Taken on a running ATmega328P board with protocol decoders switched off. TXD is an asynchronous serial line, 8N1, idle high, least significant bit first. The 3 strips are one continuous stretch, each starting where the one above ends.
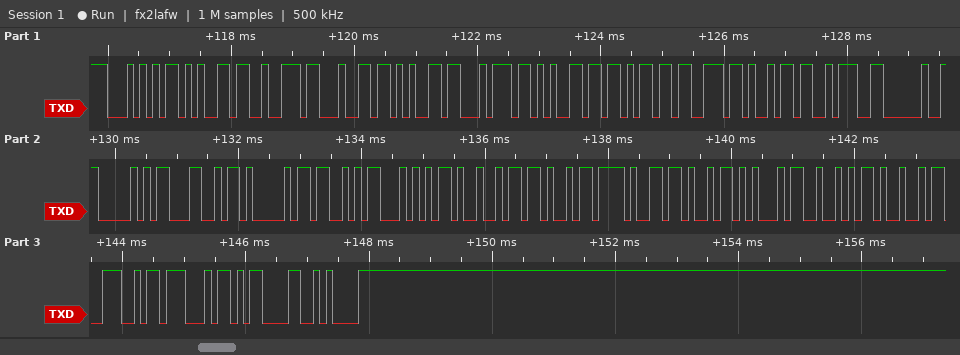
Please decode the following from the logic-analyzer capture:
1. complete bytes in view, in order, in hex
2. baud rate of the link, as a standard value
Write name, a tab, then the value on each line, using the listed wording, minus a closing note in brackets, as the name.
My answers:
complete bytes in view, in order, in hex	54 65 72 64 65 74 65 6B 73 69 3A 20 50 4C 41 53 54 49 4B 2F 4B 45 52 49 4E 47 0D 0A
baud rate of the link, as a standard value	9600 baud
